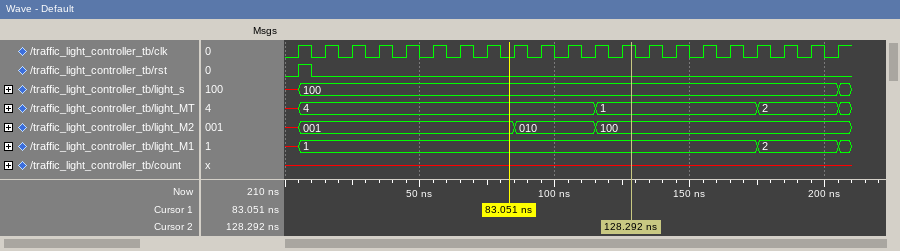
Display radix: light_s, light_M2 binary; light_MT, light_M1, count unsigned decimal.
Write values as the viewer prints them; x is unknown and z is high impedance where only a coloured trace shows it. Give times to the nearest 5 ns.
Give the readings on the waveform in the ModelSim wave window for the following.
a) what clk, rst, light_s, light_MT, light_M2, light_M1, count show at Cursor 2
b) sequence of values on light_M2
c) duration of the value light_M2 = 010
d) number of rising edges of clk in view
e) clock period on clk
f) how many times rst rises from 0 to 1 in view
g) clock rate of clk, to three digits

clk=1, rst=0, light_s=100, light_MT=1, light_M2=100, light_M1=1, count=x
x, 001, 010, 100
30 ns
21
10 ns
1
100 MHz
